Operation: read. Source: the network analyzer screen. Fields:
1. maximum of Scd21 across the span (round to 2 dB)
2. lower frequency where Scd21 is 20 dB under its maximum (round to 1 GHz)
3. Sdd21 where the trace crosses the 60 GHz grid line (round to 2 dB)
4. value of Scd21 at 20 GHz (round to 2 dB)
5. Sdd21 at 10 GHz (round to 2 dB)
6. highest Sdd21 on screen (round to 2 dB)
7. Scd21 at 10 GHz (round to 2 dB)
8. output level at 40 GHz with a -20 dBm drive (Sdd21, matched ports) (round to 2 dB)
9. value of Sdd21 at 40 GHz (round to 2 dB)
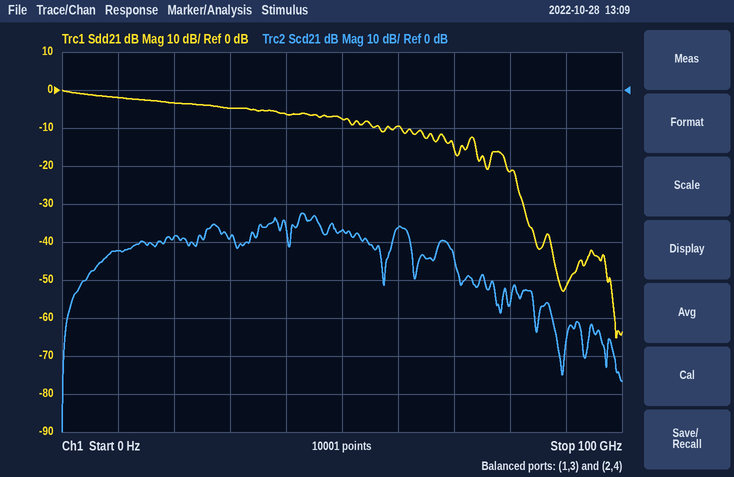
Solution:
-32 dB
3 GHz
-10 dB
-38 dB
-2 dB
0 dB
-42 dB
-26 dBm
-6 dB
